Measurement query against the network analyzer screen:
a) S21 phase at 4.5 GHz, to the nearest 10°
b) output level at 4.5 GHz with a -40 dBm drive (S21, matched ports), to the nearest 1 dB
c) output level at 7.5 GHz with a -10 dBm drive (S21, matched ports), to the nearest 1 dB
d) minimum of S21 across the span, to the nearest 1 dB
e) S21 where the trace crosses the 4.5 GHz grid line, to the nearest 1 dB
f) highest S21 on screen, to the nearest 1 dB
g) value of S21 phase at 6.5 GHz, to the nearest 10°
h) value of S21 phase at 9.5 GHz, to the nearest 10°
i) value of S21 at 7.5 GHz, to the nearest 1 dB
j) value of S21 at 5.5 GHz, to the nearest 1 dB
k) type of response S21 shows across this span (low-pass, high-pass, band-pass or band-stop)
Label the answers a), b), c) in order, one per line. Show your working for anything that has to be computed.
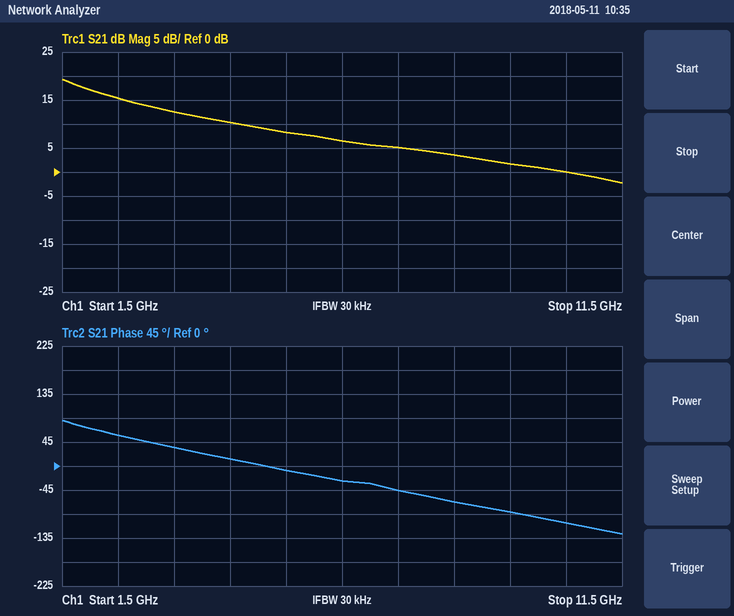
a) 10°
b) -40 dBm + (10 dB) = -30 dBm
c) -10 dBm + (5 dB) = -5 dBm
d) -2 dB
e) 10 dB
f) 19 dB
g) -30°
h) -90°
i) 5 dB
j) 8 dB
k) low-pass
